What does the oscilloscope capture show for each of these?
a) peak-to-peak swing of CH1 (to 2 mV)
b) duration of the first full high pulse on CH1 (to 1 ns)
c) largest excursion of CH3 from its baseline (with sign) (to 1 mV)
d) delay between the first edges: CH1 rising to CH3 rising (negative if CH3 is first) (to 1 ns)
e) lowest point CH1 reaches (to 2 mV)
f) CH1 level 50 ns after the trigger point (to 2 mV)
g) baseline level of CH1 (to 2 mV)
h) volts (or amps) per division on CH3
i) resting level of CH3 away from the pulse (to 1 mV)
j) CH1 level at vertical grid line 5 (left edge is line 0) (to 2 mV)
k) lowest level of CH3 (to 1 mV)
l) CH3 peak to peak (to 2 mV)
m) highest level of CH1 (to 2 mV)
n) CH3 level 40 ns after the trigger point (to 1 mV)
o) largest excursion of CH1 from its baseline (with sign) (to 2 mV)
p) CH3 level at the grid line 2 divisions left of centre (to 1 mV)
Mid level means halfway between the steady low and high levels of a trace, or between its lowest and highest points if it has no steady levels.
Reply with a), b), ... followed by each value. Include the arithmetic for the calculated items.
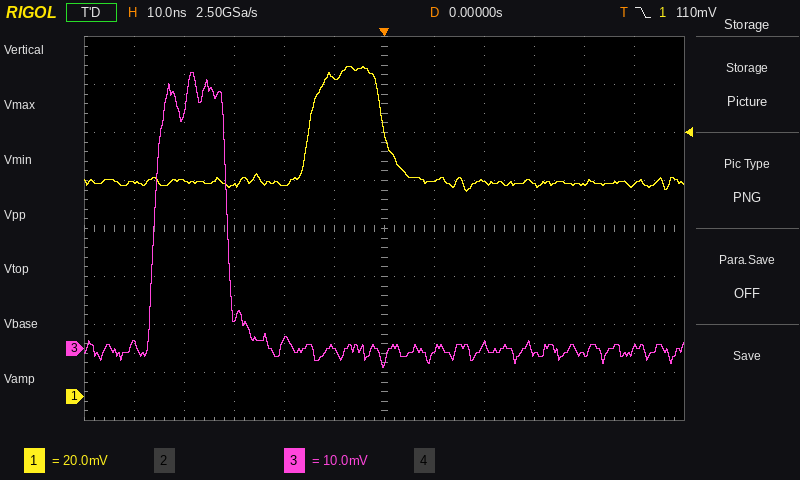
a) 138 mV − (86 mV) = 52 mV
b) 15 ns
c) +58 mV
d) -31 ns
e) 86 mV
f) 88 mV
g) 90 mV
h) 10 mV
i) 0 mV
j) 132 mV
k) -4 mV
l) 62 mV
m) 138 mV
n) -1 mV
o) 138 mV − (90 mV) = +48 mV
p) 2 mV
